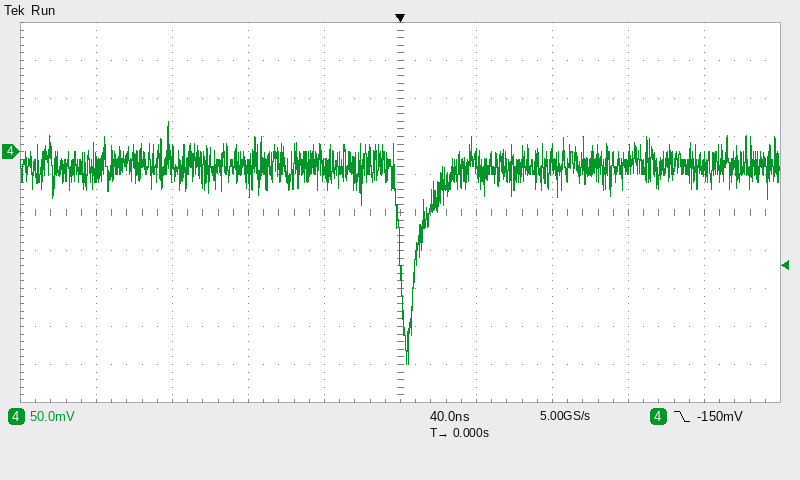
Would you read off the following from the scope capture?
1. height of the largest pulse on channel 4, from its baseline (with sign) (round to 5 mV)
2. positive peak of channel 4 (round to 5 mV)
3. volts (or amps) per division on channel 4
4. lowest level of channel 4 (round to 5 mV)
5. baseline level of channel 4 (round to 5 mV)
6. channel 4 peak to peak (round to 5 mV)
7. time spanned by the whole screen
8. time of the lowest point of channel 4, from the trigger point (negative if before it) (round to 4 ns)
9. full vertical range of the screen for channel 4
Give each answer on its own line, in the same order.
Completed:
-260 mV
40 mV
50 mV
-280 mV
-20 mV
320 mV
400 ns
+4 ns
500 mV
